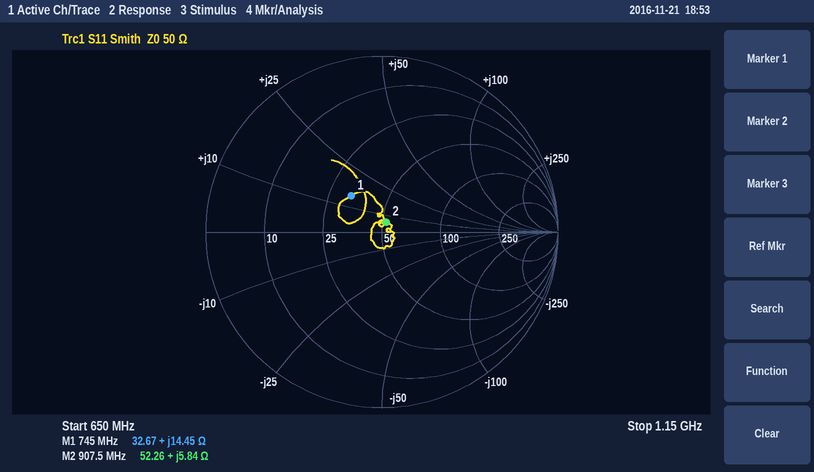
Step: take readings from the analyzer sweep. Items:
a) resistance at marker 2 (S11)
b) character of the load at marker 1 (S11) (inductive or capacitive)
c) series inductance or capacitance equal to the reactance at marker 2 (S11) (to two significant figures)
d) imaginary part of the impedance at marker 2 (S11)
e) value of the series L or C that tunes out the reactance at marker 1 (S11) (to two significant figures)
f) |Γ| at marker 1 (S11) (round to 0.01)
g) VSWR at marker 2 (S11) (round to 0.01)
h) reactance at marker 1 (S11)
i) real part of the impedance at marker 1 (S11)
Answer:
52.26 Ω
inductive
1.0 nH
+5.84 Ω
15 pF
0.27
1.13
+14.45 Ω
32.67 Ω
